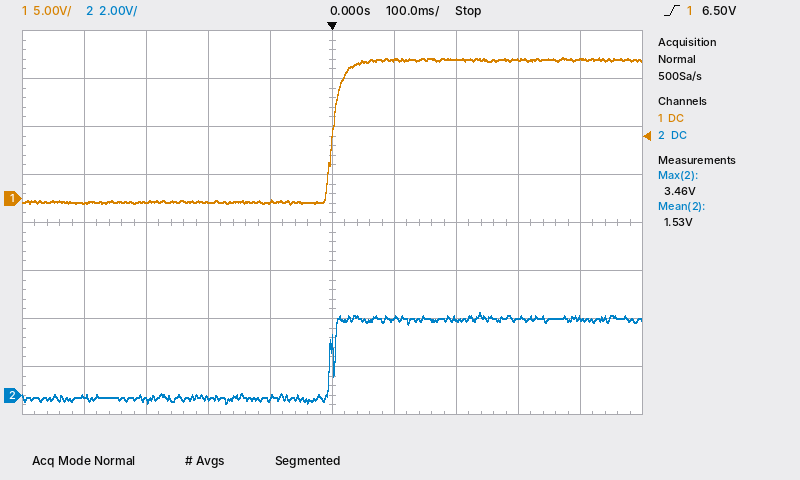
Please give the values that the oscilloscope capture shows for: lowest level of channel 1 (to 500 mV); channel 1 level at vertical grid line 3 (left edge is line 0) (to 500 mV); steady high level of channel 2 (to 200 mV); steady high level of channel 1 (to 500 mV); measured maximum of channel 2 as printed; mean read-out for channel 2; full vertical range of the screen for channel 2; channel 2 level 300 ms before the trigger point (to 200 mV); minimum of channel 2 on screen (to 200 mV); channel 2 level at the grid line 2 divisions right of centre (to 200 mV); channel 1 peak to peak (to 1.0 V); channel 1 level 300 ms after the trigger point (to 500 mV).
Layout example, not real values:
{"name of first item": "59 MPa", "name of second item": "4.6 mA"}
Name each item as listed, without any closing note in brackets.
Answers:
{"lowest level of channel 1": "-500 mV", "channel 1 level at vertical grid line 3 (left edge is line 0)": "-500 mV", "steady high level of channel 2": "3.2 V", "steady high level of channel 1": "14.5 V", "measured maximum of channel 2 as printed": "3.46 V", "mean read-out for channel 2": "1.53 V", "full vertical range of the screen for channel 2": "16 V", "channel 2 level 300 ms before the trigger point": "-200 mV", "minimum of channel 2 on screen": "-400 mV", "channel 2 level at the grid line 2 divisions right of centre": "3.2 V", "channel 1 peak to peak": "15.0 V", "channel 1 level 300 ms after the trigger point": "14.5 V"}
